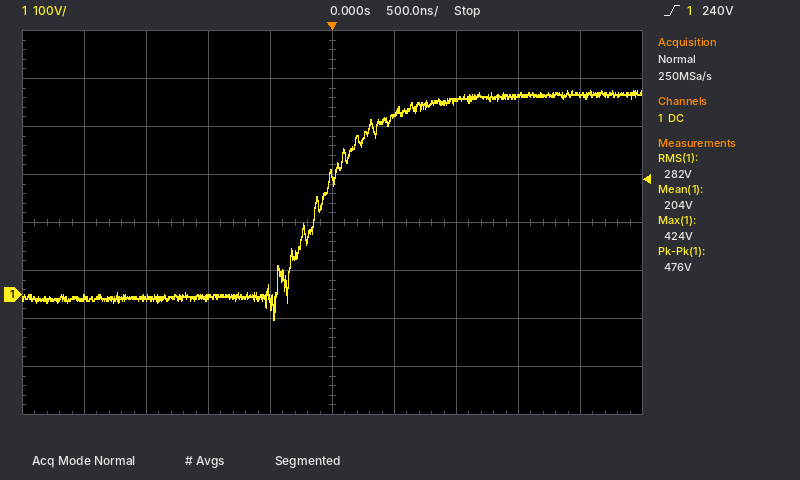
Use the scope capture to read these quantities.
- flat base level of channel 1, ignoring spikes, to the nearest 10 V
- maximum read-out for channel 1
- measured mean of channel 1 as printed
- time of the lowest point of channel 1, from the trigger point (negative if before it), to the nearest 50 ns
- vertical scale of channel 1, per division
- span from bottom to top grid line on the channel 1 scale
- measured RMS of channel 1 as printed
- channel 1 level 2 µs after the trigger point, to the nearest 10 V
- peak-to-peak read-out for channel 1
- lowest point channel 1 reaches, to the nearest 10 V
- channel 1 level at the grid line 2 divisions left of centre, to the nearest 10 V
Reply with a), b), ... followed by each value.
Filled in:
a) -10 V
b) 424 V
c) 204 V
d) -450 ns
e) 100 V
f) 800 V
g) 282 V
h) 420 V
i) 476 V
j) -50 V
k) -10 V
